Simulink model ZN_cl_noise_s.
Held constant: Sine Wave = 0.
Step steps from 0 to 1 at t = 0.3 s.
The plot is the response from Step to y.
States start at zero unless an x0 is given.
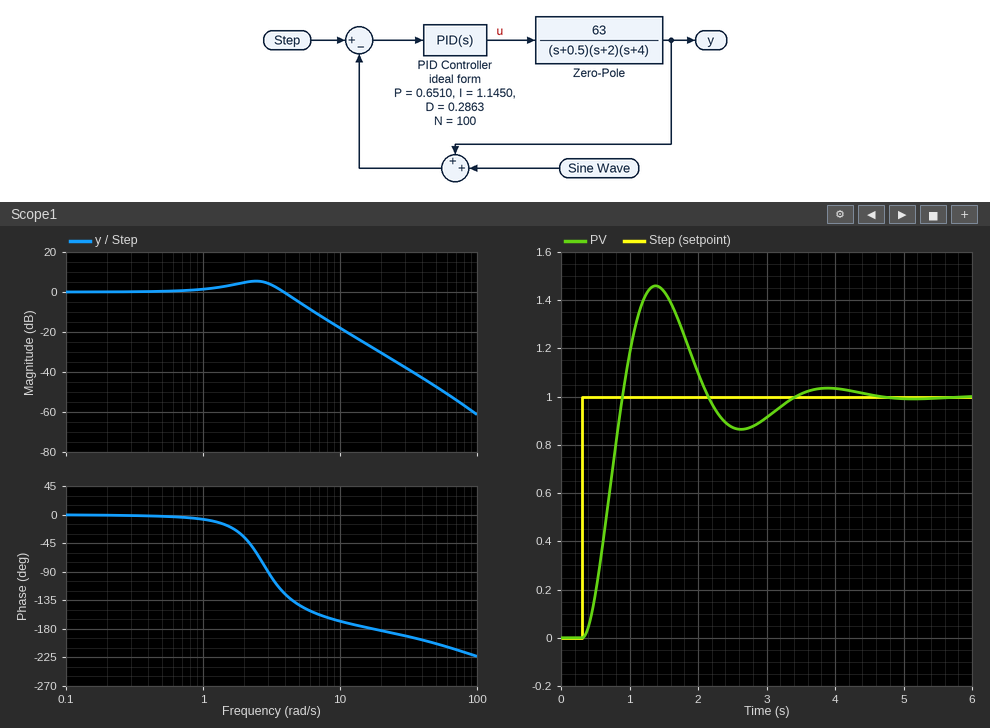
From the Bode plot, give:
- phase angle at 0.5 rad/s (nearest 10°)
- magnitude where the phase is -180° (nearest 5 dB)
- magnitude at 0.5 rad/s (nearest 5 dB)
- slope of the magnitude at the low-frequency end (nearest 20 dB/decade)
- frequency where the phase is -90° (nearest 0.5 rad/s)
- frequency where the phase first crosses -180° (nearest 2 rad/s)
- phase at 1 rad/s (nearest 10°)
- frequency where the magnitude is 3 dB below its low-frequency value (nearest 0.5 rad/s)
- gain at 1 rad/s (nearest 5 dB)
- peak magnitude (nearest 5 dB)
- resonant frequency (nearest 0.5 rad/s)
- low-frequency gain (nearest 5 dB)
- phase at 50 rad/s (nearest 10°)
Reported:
0°
-30 dB
0 dB
0 dB/decade
3.0 rad/s
18 rad/s
-10°
4.5 rad/s
0 dB
5 dB
2.5 rad/s
0 dB
-200°
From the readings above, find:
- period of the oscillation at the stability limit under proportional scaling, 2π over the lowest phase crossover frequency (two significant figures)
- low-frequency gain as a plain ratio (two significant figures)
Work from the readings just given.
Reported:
0.35 s
1.0
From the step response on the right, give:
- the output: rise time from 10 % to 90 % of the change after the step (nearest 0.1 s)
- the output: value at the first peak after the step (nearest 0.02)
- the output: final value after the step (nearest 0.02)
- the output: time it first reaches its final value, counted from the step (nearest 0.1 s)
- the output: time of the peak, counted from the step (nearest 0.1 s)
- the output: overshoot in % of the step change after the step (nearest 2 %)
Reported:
0.4 s
1.46
1.00
0.6 s
1.1 s
46 %
